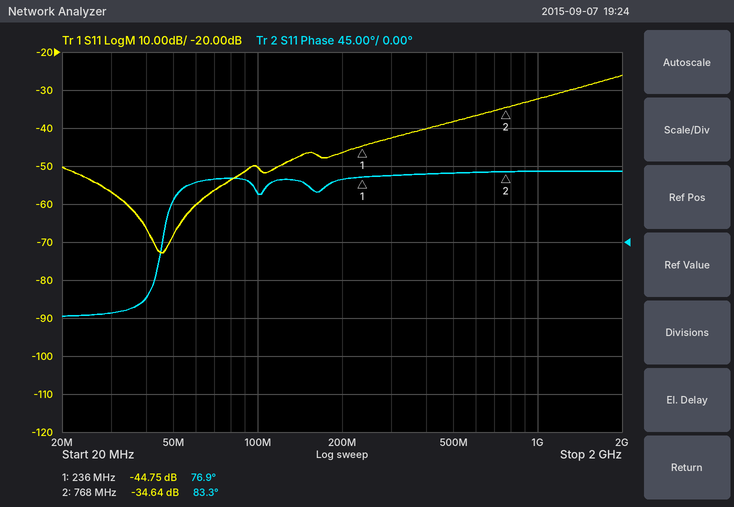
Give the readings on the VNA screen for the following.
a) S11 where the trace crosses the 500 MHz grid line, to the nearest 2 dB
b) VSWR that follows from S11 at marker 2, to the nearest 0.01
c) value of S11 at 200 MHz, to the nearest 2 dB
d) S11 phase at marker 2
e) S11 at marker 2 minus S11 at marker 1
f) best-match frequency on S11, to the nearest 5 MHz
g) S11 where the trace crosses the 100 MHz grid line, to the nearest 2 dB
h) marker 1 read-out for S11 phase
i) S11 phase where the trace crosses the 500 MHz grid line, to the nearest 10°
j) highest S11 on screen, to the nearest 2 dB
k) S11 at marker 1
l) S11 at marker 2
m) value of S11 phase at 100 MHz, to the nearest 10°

-38 dB
1.04
-46 dB
83.3°
10.11 dB
45 MHz
-50 dB
76.9°
80°
-26 dB
-44.75 dB
-34.64 dB
60°
